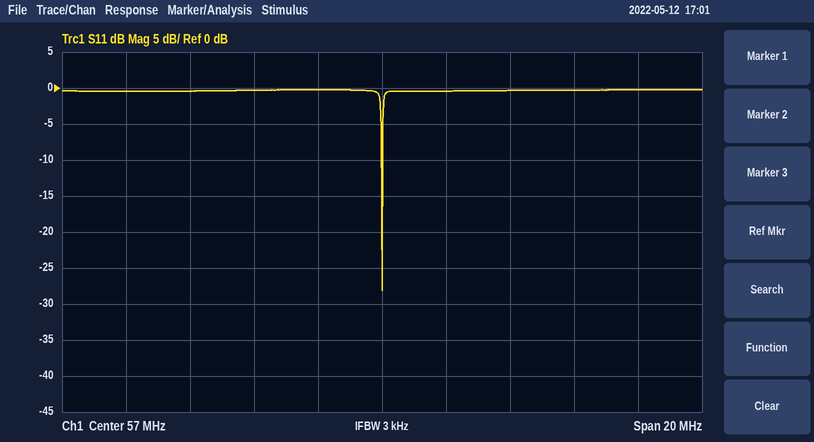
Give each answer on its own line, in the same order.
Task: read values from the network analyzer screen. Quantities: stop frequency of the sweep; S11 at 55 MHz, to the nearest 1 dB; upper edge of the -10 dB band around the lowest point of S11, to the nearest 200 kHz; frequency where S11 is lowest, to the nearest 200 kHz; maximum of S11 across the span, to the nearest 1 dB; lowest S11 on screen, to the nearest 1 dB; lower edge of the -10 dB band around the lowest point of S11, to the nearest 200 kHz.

67 MHz
0 dB
57.0 MHz
57.0 MHz
0 dB
-28 dB
57.0 MHz
